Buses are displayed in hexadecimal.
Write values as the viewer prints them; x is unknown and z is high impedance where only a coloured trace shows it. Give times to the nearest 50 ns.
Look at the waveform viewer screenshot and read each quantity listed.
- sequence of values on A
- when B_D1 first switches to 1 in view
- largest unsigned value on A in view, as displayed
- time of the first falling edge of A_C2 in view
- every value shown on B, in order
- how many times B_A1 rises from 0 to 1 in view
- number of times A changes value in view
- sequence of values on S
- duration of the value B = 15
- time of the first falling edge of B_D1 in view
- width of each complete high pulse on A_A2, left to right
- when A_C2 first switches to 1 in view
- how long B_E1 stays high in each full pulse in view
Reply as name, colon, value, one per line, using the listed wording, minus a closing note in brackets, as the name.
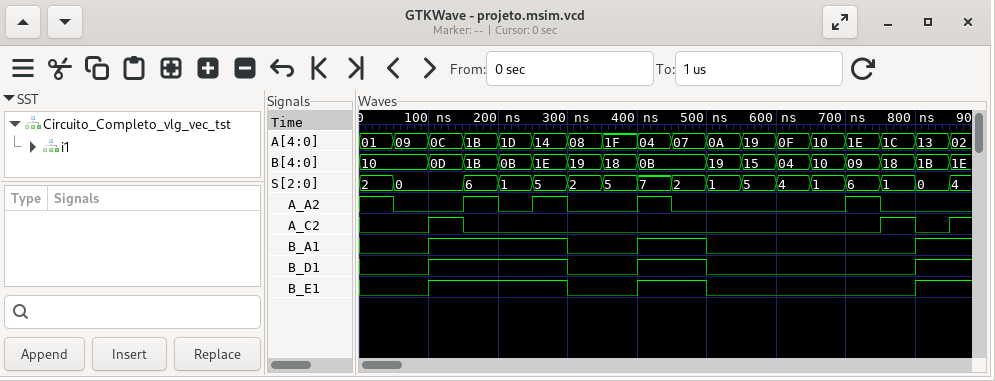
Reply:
sequence of values on A: 01, 09, 0C, 1B, 1D, 14, 08, 1F, 04, 07, 0A, 19, 0F, 10, 1E, 1C, 13, 02
when B_D1 first switches to 1 in view: 100 ns
largest unsigned value on A in view, as displayed: 1F
time of the first falling edge of A_C2 in view: 150 ns
every value shown on B, in order: 10, 0D, 1B, 0B, 1E, 19, 18, 0B, 19, 15, 04, 10, 09, 18, 1B, 1E
how many times B_A1 rises from 0 to 1 in view: 3
number of times A changes value in view: 17
sequence of values on S: 2, 0, 6, 1, 5, 2, 5, 7, 2, 1, 5, 4, 1, 6, 1, 0, 4
duration of the value B = 15: 50 ns
time of the first falling edge of B_D1 in view: 300 ns
width of each complete high pulse on A_A2, left to right: 50 ns, 50 ns, 50 ns, 50 ns
when A_C2 first switches to 1 in view: 100 ns
how long B_E1 stays high in each full pulse in view: 200 ns, 100 ns
